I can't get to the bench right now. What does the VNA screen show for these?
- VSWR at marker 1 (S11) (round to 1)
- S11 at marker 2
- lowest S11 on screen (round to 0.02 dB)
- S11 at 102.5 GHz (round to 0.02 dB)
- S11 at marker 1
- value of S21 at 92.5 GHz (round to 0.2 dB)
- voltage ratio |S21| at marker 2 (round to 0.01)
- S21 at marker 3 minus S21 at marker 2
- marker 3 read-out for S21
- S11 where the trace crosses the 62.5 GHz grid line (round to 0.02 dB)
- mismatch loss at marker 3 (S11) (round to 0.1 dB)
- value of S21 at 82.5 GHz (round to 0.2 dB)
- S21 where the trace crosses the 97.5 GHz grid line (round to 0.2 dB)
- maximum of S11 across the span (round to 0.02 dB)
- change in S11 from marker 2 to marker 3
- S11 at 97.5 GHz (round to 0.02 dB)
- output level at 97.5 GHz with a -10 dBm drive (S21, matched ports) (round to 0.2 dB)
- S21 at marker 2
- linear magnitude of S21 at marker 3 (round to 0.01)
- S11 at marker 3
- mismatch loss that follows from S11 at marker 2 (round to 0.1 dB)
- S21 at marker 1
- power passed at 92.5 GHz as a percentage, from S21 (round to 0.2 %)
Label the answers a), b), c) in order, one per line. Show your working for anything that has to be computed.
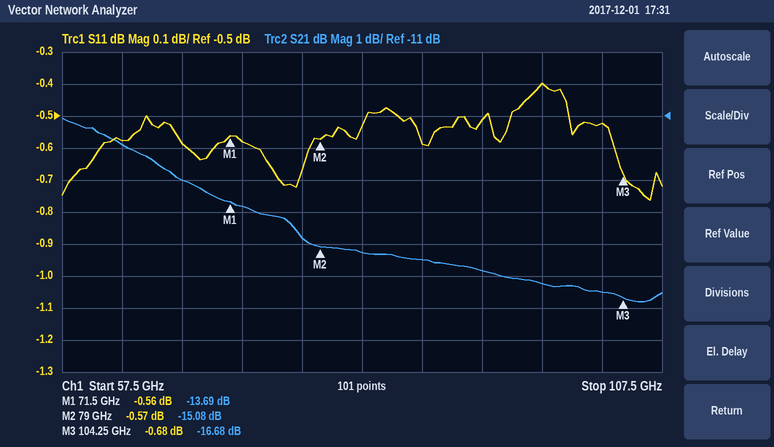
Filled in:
a) (1 + 0.9376)/(1 − 0.9376) ≈ 31
b) -0.57 dB
c) -0.76 dB
d) -0.52 dB
e) -0.56 dB
f) -15.8 dB
g) 10^(-15.08/20) ≈ 0.18
h) -16.68 − (-15.08) = -1.60 dB
i) -16.68 dB
j) -0.58 dB
k) −10 log10(1 − 10^(-0.68/10)) ≈ 8.4 dB
l) -15.2 dB
m) -16.2 dB
n) -0.40 dB
o) -0.68 − (-0.57) = -0.11 dB
p) -0.40 dB
q) -10 dBm + (-16.2 dB) = -26.2 dBm
r) -15.08 dB
s) 10^(-16.68/20) ≈ 0.15
t) -0.68 dB
u) −10 log10(1 − 10^(-0.57/10)) ≈ 9.1 dB
v) -13.69 dB
w) 10^(-15.8/10) ≈ 2.6 %
